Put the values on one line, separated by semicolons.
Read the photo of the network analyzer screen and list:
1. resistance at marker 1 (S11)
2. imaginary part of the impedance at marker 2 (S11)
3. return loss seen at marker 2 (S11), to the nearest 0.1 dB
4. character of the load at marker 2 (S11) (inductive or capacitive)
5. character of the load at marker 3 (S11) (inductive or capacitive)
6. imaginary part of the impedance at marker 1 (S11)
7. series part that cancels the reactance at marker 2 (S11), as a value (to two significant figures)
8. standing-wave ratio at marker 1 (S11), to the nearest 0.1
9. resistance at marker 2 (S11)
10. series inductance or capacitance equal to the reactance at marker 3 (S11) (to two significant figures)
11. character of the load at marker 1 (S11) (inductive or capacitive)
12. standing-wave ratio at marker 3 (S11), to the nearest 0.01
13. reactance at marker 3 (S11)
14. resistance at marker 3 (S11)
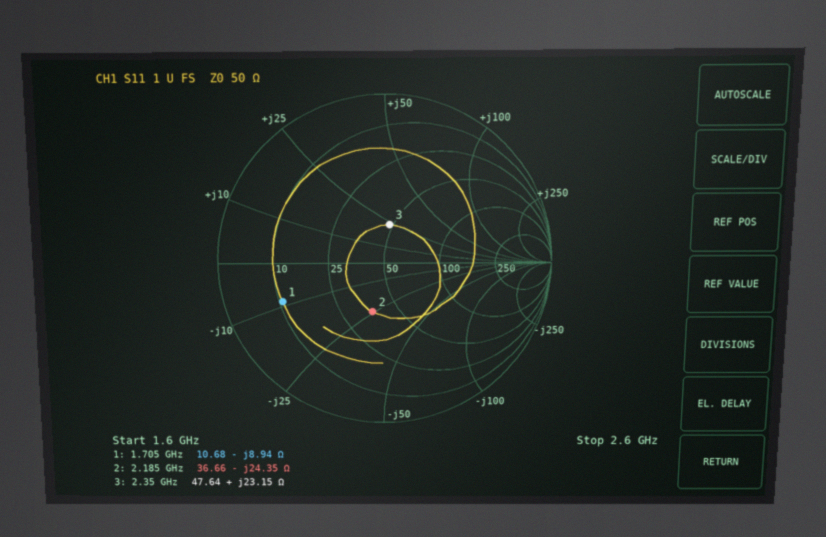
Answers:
10.68 Ω; -24.35 Ω; 10.2 dB; capacitive; inductive; -8.94 Ω; 1.8 nH; 4.8; 36.66 Ω; 1.6 nH; capacitive; 1.60; +23.15 Ω; 47.64 Ω
